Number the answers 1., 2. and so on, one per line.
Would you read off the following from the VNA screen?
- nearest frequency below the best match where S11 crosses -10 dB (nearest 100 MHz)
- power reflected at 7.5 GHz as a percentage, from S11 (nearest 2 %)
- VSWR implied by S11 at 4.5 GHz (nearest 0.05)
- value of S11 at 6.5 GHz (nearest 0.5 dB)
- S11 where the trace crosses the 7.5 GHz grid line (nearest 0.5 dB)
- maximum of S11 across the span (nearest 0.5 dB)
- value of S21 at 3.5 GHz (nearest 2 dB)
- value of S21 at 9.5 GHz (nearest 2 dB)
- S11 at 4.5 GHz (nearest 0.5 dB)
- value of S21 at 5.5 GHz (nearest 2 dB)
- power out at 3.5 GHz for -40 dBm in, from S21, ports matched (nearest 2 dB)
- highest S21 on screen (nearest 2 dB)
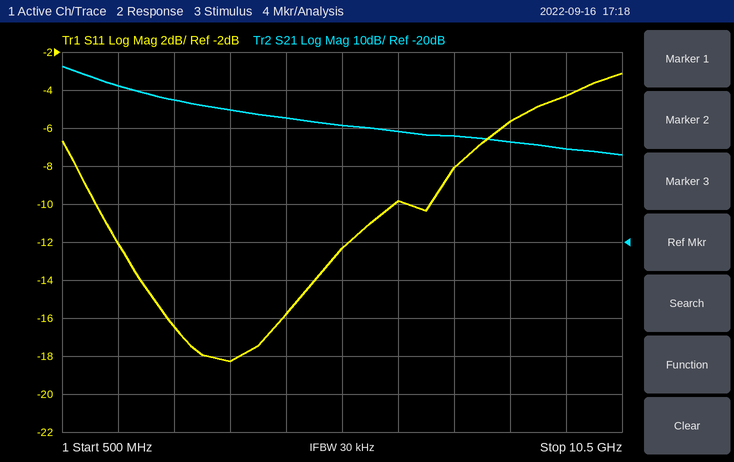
1. 1.1 GHz
2. 16 %
3. 1.40
4. -10.0 dB
5. -8.0 dB
6. -3.0 dB
7. 14 dB
8. 4 dB
9. -16.0 dB
10. 10 dB
11. -26 dBm
12. 26 dB
